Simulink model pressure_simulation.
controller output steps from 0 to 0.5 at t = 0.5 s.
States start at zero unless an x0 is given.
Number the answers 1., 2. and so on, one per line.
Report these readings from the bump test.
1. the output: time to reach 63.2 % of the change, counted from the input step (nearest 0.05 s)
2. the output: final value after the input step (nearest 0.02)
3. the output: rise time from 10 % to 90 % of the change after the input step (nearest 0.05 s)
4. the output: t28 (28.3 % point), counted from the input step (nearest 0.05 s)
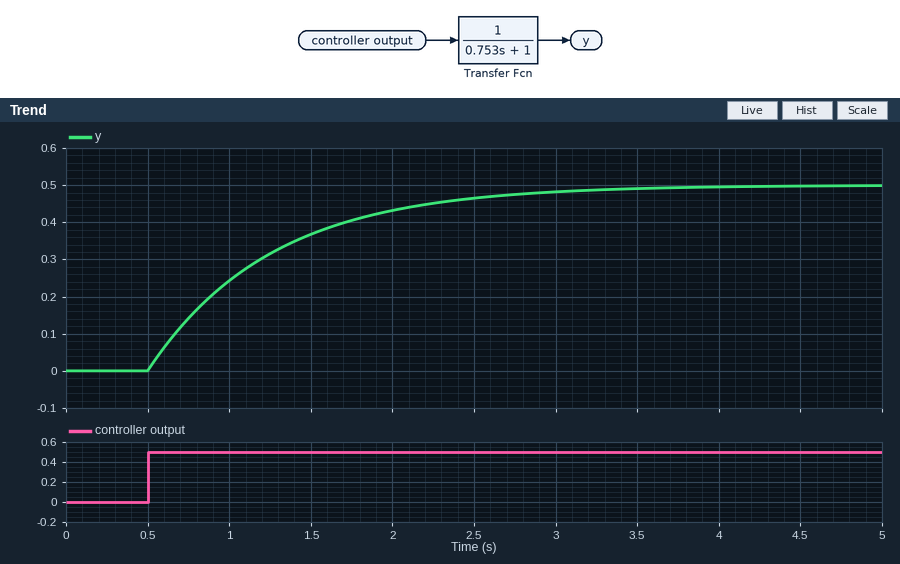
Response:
1. 0.75 s
2. 0.50
3. 1.65 s
4. 0.25 s
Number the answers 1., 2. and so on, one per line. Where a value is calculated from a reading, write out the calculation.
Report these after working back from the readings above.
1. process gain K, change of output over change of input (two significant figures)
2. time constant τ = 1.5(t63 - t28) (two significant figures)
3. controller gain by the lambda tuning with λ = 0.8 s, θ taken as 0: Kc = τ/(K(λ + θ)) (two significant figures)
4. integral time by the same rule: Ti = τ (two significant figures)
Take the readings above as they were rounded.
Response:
1. (0.5 - 0) / 0.5 = 1.0
2. 1.5 × (0.75 - 0.25) = 0.75 s
3. 0.75 / (1 × (0.8 + 0)) = 0.94
4. 0.75 s
